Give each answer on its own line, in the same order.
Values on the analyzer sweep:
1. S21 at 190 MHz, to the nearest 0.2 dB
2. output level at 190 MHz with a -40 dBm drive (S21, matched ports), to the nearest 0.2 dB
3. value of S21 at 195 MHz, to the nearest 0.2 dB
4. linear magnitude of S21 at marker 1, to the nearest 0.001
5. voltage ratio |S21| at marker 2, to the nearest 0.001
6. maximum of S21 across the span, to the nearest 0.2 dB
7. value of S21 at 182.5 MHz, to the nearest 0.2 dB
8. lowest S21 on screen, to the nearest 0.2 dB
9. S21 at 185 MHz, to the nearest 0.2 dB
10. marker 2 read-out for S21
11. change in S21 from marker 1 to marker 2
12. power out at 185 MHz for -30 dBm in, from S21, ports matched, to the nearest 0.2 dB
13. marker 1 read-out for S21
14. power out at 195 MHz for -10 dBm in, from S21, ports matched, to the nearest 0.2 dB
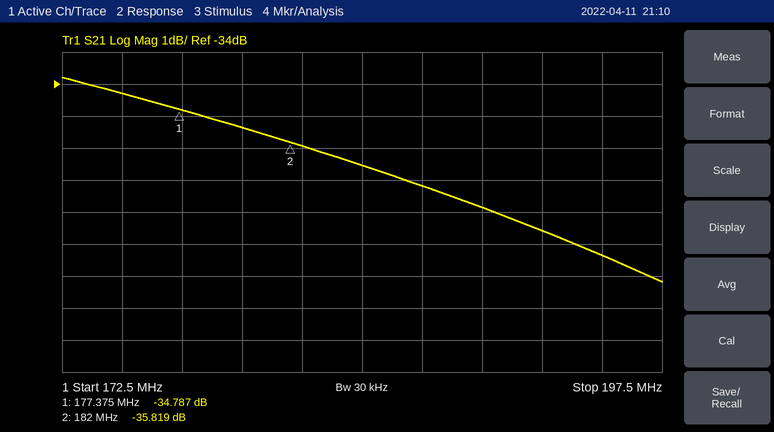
-37.8 dB
-77.8 dBm
-39.4 dB
0.018
0.016
-33.8 dB
-36.0 dB
-40.2 dB
-36.6 dB
-35.819 dB
-1.032 dB
-66.6 dBm
-34.787 dB
-49.4 dBm
